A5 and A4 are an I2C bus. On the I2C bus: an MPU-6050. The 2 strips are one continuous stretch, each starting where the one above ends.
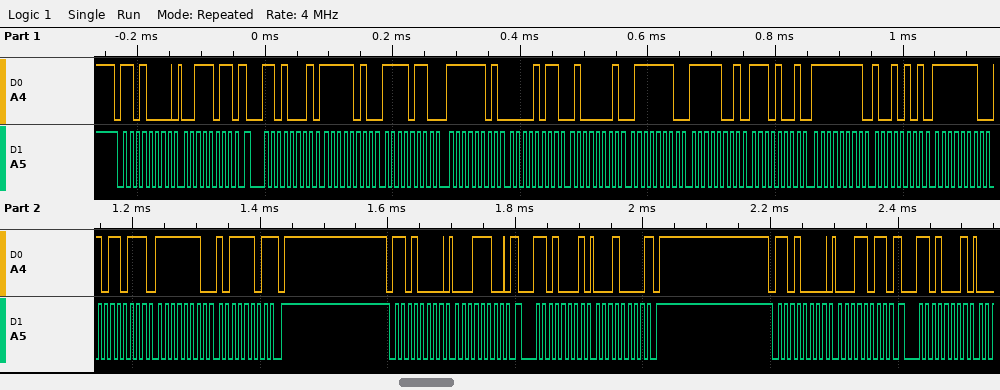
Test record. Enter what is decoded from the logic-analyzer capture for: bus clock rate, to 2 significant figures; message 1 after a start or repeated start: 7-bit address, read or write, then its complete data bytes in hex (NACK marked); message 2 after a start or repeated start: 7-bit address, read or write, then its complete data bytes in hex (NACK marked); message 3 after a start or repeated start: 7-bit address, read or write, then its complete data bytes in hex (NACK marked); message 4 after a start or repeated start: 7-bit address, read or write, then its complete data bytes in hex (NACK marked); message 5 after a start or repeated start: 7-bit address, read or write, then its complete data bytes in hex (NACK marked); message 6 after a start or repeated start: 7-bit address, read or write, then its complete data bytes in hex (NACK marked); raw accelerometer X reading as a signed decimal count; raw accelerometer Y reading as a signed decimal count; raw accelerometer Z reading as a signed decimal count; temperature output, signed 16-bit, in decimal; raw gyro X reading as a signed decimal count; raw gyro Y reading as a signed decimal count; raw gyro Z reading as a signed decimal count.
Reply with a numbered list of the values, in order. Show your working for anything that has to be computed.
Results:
1. 100 kHz
2. 0x68 write: 3B
3. 0x68 read: FA F6 FD 0B 41 7E F9 E9 FF 95 FE B7 FE BD NACK
4. 0x68 write: 1C
5. 0x68 read: 10 NACK
6. 0x68 write: 1B
7. 0x68 read
8. 0xFAF6 = -1290
9. 0xFD0B = -757
10. 0x417E = 16766
11. 0xF9E9 = -1559
12. 0xFF95 = -107
13. 0xFEB7 = -329
14. 0xFEBD = -323
